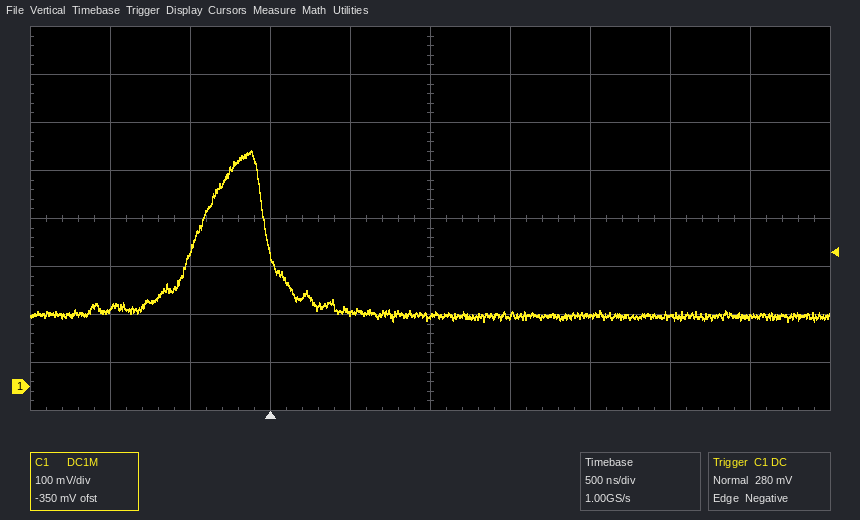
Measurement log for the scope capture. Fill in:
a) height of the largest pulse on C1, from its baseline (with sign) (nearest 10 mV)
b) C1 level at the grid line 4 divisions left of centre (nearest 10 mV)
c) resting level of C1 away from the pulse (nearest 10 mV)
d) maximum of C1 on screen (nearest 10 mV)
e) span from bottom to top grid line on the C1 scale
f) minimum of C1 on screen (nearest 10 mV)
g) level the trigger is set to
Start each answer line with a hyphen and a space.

- +340 mV
- 160 mV
- 150 mV
- 490 mV
- 800 mV
- 140 mV
- 280 mV
